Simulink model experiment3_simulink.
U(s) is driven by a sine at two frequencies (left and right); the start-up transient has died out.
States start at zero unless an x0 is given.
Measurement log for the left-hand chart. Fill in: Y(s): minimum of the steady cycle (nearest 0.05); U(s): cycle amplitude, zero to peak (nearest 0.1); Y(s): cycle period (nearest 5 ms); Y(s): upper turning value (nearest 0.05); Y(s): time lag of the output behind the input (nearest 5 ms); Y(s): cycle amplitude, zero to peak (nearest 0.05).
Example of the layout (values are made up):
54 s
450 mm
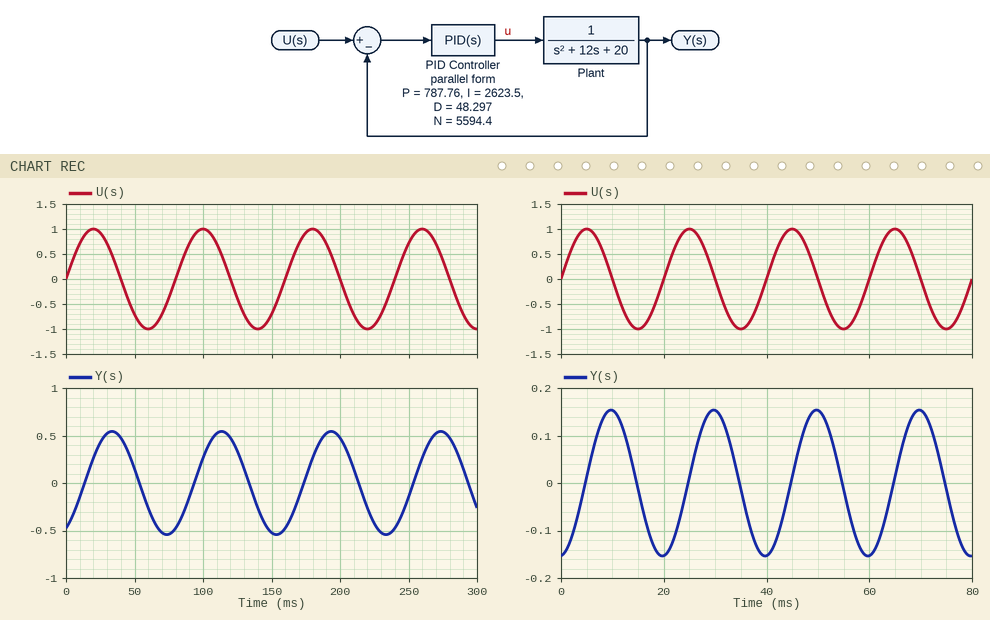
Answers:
-0.55
1.0
80 ms
0.55
15 ms
0.55
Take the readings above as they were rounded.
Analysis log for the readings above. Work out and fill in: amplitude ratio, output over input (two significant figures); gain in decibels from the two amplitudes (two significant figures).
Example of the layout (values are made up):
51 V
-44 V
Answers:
0.55
-5.2 dB
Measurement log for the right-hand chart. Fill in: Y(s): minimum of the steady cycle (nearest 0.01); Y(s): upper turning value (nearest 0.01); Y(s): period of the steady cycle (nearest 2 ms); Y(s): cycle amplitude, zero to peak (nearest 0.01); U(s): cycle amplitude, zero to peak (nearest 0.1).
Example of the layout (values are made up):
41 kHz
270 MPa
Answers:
-0.15
0.15
20 ms
0.15
1.0
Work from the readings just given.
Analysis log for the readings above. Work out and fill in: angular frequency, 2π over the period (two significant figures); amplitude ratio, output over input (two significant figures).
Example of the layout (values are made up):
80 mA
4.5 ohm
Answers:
0.31 rad/ms
0.15
